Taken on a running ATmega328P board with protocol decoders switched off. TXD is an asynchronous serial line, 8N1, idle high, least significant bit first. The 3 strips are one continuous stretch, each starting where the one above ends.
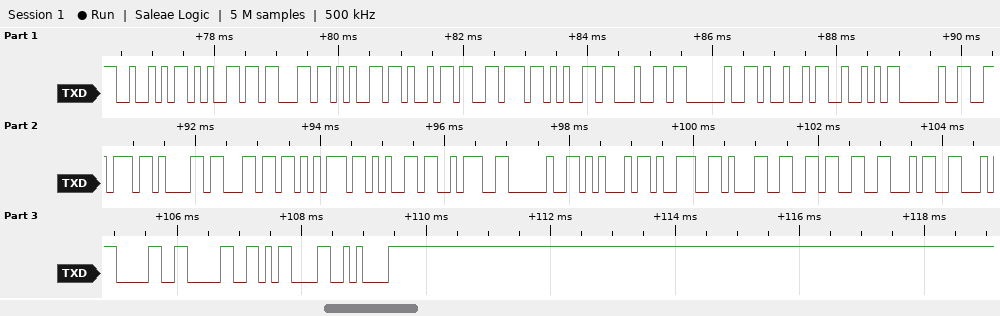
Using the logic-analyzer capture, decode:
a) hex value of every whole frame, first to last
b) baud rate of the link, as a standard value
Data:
0x52 0x65 0x63 0x65 0x69 0x76 0x65 0x64 0x20 0x49 0x52 0x20 0x76 0x61 0x6C 0x75 0x65 0x3A 0x20 0x45 0x39 0x31 0x36 0x46 0x46 0x30 0x30 0x0D 0x0A
9600 baud
